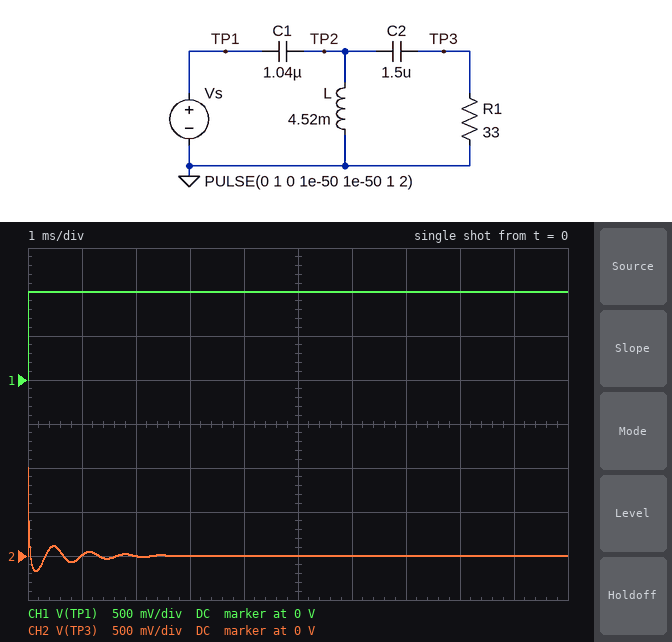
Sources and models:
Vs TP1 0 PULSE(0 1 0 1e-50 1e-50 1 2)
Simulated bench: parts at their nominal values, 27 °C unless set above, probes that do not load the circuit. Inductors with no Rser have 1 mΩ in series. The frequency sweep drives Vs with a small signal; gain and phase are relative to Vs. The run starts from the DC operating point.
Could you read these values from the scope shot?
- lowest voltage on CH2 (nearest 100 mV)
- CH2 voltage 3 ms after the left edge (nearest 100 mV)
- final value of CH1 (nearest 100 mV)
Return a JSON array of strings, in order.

["-200 mV", "0 V", "1.0 V"]
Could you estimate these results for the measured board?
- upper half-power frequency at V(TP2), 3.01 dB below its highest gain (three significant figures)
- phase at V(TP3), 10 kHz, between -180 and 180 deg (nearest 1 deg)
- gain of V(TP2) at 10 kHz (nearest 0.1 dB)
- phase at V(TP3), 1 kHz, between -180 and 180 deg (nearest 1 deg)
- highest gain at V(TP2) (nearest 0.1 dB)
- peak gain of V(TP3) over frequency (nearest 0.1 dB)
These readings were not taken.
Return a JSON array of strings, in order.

["1.85 kHz", "39 deg", "-1.3 dB", "-115 deg", "4.9 dB", "0 dB"]
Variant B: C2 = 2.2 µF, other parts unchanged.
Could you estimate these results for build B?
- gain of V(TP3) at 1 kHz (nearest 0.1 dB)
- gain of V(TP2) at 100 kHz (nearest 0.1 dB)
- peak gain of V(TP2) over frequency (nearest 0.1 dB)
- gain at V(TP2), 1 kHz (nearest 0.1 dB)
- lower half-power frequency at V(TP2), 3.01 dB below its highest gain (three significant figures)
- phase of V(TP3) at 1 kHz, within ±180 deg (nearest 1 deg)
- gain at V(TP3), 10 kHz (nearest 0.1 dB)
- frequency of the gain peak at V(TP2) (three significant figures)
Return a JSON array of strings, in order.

["-16.4 dB", "0 dB", "0.2 dB", "-8.8 dB", "1.21 kHz", "-131 deg", "-1.3 dB", "1.45 kHz"]
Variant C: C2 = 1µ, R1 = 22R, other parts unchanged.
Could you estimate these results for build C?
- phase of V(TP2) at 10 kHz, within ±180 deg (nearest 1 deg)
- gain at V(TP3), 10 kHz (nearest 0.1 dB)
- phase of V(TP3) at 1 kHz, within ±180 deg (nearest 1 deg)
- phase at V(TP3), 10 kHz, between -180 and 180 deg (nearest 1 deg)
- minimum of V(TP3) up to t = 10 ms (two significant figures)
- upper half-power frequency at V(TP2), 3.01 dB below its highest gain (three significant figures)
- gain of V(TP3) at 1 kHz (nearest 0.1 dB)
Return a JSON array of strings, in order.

["20 deg", "-4.5 dB", "-100 deg", "56 deg", "-110 mV", "1.78 kHz", "-28.0 dB"]
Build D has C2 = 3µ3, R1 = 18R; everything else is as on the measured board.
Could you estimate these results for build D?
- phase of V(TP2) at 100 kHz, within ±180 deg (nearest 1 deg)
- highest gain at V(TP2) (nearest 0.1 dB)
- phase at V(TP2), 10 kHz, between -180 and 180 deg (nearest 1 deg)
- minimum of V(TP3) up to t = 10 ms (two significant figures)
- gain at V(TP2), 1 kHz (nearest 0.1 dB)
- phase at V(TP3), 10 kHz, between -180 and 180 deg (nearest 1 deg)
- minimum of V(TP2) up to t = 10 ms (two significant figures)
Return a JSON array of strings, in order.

["5 deg", "0 dB", "34 deg", "-89 mV", "-5.6 dB", "49 deg", "-170 mV"]
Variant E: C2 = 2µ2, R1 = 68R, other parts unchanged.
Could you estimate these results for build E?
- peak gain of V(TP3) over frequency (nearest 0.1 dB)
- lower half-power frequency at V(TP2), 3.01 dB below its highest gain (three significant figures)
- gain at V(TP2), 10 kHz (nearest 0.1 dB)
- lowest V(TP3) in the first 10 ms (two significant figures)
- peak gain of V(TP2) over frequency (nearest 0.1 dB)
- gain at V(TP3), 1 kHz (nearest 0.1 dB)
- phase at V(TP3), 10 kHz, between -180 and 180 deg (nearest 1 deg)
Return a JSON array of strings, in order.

["0.3 dB", "1.48 kHz", "0 dB", "-330 mV", "1.1 dB", "-14.0 dB", "19 deg"]
